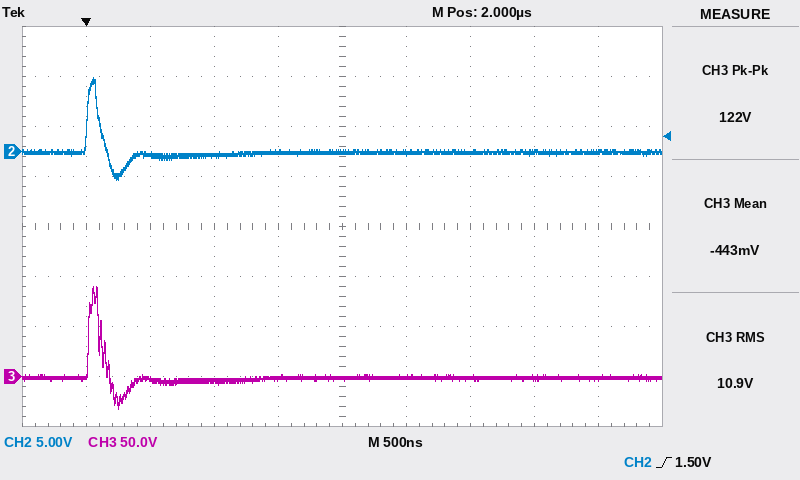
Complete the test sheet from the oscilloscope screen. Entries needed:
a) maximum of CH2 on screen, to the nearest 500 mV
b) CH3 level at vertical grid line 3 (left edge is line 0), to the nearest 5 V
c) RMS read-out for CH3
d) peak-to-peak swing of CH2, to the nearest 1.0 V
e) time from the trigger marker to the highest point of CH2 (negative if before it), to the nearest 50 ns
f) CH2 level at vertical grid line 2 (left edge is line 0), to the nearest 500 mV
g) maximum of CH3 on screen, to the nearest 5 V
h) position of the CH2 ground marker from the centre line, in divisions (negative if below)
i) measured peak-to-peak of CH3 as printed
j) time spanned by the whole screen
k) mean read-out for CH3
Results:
7.5 V
-5 V
10.9 V
10.0 V
+50 ns
-500 mV
90 V
+1.5 div
122 V
5 µs
-443 mV
